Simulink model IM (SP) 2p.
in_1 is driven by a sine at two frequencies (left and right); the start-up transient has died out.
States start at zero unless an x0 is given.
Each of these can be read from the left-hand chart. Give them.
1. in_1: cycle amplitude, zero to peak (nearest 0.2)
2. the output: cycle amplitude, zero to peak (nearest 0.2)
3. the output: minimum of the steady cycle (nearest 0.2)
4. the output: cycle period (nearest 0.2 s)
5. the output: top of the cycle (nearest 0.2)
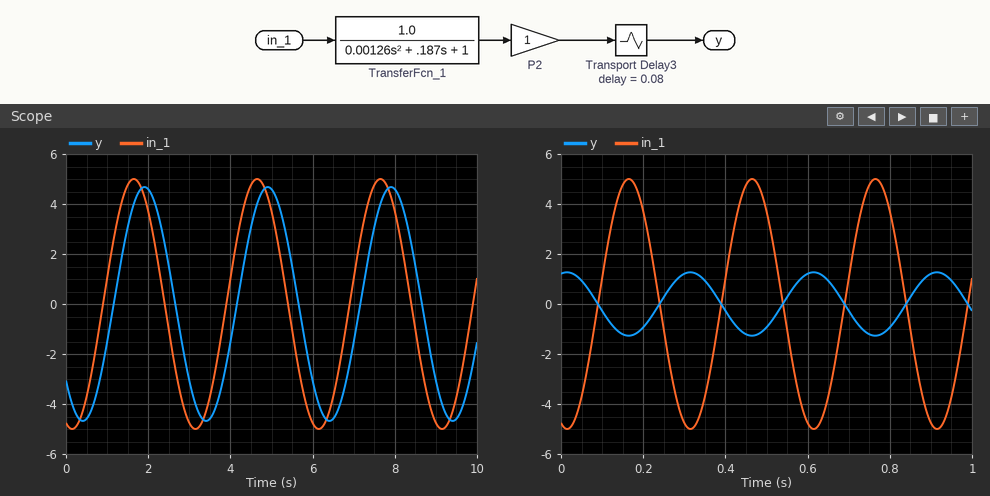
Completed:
5.0
4.6
-4.6
3.0 s
4.6
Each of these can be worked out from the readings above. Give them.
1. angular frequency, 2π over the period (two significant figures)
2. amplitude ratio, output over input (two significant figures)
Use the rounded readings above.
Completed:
2.1 rad/s
0.92
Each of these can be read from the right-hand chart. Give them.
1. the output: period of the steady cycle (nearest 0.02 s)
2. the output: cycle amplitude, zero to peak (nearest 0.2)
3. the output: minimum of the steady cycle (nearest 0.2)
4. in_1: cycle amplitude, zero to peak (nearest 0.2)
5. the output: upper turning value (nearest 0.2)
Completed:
0.30 s
1.2
-1.2
5.0
1.2
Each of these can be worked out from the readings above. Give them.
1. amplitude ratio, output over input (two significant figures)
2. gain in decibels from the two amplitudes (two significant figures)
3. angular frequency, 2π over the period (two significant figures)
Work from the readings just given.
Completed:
0.24
-12 dB
21 rad/s
